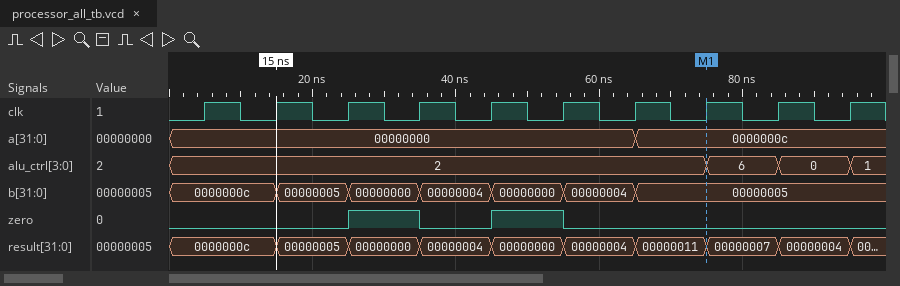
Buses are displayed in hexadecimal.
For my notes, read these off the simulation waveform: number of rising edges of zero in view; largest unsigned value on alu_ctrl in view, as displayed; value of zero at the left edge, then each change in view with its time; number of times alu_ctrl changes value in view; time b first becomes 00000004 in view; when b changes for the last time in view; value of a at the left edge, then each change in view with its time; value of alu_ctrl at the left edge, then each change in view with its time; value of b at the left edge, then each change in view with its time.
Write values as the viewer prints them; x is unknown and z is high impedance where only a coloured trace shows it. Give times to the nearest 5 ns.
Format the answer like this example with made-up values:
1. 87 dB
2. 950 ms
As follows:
1. 2
2. 6
3. 0, 1 at 25 ns, 0 at 35 ns, 1 at 45 ns, 0 at 55 ns
4. 3
5. 35 ns
6. 65 ns
7. 00000000, 0000000c at 65 ns
8. 2, 6 at 75 ns, 0 at 85 ns, 1 at 95 ns
9. 0000000c, 00000005 at 15 ns, 00000000 at 25 ns, 00000004 at 35 ns, 00000000 at 45 ns, 00000004 at 55 ns, 00000005 at 65 ns
